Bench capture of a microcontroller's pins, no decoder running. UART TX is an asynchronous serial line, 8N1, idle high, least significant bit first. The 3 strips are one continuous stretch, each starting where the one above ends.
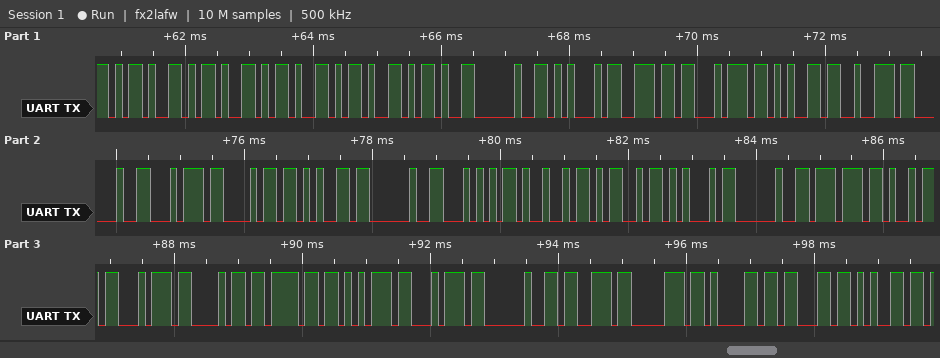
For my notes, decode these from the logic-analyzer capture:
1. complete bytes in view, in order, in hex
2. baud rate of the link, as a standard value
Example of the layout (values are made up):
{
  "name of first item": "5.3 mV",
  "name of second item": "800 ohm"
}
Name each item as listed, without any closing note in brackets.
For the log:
{
  "complete bytes in view, in order, in hex": "2D 2D 2D 2D 2D 20 45 6E 74 65 72 20 74 68 65 20 54 49 4D 45 20 77 69 74 68 6F 75 74 20 73 70 61 63 65",
  "baud rate of the link, as a standard value": "9600 baud"
}
